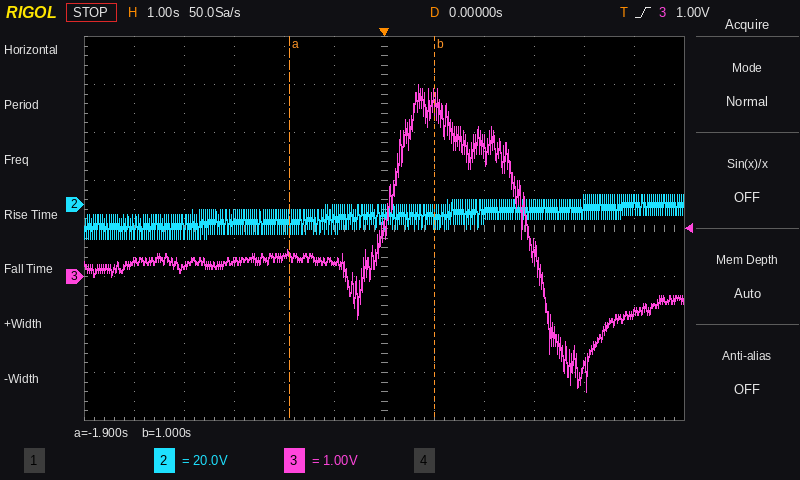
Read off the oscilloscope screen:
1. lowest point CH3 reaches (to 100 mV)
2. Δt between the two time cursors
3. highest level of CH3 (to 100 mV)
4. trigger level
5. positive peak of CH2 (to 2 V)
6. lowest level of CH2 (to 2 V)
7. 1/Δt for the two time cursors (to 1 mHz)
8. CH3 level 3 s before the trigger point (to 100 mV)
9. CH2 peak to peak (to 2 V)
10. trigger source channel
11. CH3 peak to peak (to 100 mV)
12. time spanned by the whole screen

-2.4 V
2.9 s
4.0 V
1.00 V
4 V
-14 V
345 mHz
300 mV
18 V
CH3
6.4 V
12 s
